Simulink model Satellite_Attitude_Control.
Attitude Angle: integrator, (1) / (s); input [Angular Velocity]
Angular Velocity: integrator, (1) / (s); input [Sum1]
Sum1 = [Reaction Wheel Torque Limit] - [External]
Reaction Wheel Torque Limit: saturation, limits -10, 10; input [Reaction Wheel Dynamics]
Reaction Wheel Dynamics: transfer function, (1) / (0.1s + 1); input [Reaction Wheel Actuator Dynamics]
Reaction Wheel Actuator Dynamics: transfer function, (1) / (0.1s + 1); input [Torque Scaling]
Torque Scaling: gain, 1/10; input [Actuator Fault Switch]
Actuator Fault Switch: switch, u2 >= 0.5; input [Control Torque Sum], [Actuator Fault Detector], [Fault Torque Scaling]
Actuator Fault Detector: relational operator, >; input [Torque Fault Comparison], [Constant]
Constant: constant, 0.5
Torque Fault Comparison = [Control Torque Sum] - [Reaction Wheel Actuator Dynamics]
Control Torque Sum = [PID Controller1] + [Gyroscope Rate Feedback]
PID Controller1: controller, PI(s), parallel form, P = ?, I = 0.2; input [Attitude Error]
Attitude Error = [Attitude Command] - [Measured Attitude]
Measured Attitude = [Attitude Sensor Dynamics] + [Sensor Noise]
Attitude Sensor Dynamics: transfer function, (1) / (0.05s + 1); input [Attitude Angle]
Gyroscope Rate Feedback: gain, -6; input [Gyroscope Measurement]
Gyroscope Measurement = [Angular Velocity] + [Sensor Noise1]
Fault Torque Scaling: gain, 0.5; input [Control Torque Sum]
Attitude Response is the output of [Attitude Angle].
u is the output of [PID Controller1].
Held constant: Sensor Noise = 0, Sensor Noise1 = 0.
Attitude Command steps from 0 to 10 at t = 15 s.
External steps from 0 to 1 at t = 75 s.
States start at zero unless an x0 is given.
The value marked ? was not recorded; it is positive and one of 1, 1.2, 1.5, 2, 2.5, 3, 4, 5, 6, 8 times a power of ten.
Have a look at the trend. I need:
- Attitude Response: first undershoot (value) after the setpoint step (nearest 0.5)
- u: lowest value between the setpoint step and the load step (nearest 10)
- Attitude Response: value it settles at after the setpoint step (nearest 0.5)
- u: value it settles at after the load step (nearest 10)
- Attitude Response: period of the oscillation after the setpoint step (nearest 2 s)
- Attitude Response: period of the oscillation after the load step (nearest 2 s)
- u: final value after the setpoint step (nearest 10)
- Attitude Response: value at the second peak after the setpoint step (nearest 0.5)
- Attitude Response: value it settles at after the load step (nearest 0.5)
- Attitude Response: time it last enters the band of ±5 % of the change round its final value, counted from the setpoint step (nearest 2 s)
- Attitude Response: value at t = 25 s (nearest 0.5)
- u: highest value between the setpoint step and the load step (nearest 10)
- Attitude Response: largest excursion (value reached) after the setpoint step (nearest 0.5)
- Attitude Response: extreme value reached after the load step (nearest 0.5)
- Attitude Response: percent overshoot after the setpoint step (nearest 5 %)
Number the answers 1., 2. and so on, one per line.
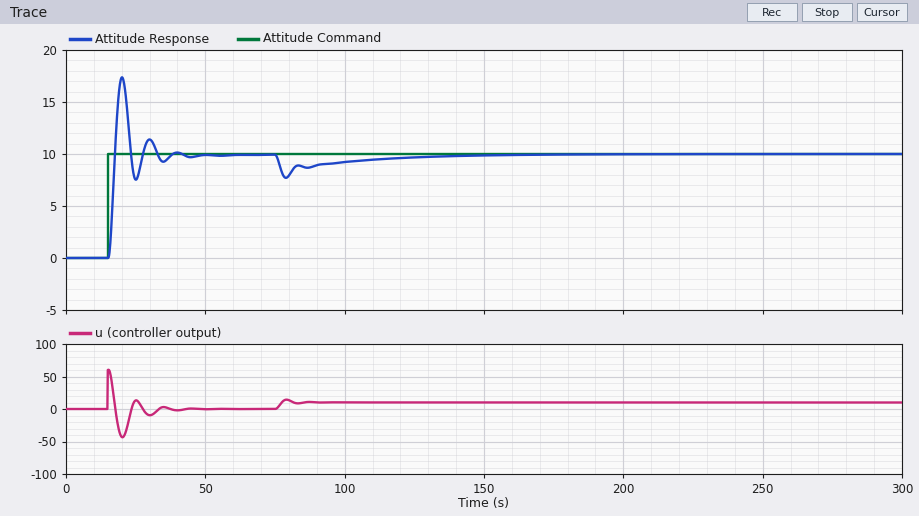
1. 7.5
2. -40
3. 10.0
4. 10
5. 10 s
6. 8 s
7. 0
8. 11.5
9. 10.0
10. 22 s
11. 7.5
12. 60
13. 17.5
14. 7.5
15. 75 %
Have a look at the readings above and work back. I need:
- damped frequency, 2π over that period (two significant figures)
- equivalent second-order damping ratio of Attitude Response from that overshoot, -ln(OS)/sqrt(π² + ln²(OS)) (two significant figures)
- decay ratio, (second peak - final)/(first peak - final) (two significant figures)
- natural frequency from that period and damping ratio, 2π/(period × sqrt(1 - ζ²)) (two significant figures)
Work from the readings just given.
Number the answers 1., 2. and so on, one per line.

1. 0.63 rad/s
2. 0.091
3. 0.20
4. 0.63 rad/s
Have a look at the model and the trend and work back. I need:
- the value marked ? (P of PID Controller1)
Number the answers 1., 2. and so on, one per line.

1. 6
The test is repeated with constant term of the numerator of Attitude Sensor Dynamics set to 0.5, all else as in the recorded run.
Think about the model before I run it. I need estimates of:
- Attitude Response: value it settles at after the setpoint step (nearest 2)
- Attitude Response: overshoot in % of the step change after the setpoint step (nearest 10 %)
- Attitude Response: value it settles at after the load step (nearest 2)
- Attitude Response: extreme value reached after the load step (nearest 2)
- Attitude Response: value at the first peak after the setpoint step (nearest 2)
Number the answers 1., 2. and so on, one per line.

1. 20
2. 50 %
3. 20
4. 16
5. 30
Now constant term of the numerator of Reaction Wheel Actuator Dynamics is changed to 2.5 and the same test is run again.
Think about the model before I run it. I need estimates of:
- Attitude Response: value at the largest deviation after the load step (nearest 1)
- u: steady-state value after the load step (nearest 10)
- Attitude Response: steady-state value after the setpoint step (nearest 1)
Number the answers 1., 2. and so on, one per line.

1. 9
2. 0
3. 10
